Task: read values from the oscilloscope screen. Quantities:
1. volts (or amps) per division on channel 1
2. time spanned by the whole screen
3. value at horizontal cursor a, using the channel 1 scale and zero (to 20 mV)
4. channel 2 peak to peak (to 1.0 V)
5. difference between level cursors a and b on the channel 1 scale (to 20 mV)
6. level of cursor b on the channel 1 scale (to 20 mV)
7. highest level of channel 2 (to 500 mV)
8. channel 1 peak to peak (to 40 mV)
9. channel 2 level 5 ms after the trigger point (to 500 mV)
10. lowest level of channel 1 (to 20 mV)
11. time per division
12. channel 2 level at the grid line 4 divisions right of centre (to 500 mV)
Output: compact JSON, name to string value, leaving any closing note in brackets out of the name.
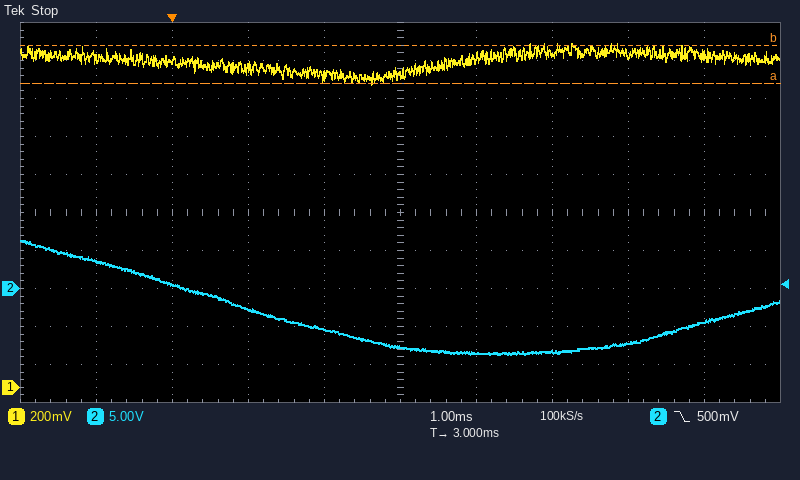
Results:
{"volts (or amps) per division on channel 1": "200 mV", "time spanned by the whole screen": "10 ms", "value at horizontal cursor a, using the channel 1 scale and zero": "1.60 V", "channel 2 peak to peak": "15.0 V", "difference between level cursors a and b on the channel 1 scale": "200 mV", "level of cursor b on the channel 1 scale": "1.80 V", "highest level of channel 2": "6.5 V", "channel 1 peak to peak": "200 mV", "channel 2 level 5 ms after the trigger point": "-8.5 V", "lowest level of channel 1": "1.60 V", "time per division": "1 ms", "channel 2 level at the grid line 4 divisions right of centre": "-4.5 V"}
